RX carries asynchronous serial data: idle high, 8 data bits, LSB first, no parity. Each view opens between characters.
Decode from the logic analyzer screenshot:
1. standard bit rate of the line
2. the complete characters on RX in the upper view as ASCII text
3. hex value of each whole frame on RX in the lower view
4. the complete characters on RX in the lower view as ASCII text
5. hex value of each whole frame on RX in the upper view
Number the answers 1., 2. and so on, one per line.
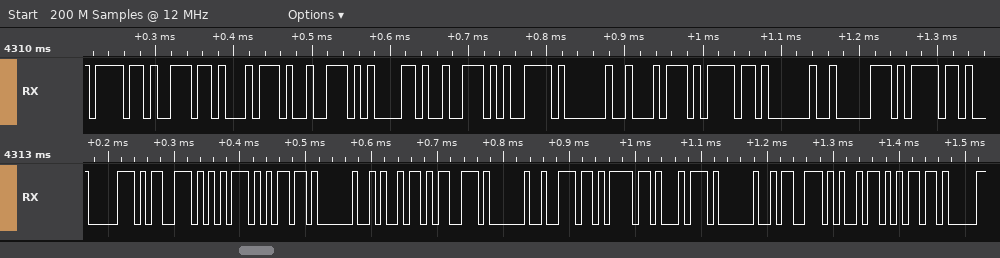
1. 115200 baud
2. "ontrary to po"
3. 70, 73, 75, 6D, 20, 69, 73, 20, 6E, 6F, 74, 20, 73, 69, 6D
4. "psum is not sim"
5. 6F, 6E, 74, 72, 61, 72, 79, 20, 74, 6F, 20, 70, 6F
